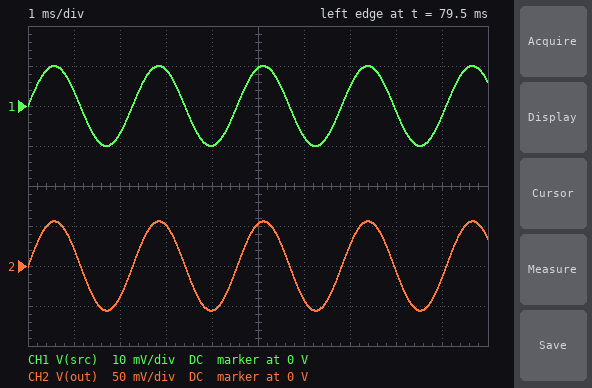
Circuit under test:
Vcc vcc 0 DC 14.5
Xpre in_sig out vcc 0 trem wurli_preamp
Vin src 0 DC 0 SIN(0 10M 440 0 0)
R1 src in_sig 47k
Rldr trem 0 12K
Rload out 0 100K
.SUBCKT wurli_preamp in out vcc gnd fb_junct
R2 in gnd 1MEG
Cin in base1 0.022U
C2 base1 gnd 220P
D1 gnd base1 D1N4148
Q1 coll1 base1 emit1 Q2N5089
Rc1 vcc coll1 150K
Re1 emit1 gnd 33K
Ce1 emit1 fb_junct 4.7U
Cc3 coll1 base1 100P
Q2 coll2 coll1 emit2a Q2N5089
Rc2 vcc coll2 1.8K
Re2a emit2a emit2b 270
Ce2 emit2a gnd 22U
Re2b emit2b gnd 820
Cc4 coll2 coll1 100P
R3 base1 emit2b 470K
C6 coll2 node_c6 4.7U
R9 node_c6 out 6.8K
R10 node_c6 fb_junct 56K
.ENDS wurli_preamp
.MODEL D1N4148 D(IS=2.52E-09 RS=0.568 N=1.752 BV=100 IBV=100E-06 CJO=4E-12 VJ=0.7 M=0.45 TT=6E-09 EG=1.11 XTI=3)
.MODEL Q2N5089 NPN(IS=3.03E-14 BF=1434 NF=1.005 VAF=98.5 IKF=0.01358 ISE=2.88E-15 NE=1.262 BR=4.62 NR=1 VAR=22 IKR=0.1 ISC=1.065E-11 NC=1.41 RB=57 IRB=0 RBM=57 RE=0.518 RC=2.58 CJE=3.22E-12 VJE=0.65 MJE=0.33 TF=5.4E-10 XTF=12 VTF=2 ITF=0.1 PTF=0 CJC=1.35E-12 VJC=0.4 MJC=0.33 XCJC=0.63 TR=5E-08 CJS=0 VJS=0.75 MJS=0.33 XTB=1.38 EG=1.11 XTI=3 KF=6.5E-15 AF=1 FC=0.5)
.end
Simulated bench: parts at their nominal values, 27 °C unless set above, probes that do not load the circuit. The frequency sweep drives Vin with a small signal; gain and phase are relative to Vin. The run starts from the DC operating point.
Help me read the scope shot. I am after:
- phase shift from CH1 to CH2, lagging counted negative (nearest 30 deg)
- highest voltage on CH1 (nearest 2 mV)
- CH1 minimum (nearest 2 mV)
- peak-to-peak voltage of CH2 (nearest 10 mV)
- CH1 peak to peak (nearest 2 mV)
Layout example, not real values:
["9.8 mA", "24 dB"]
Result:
["0 deg", "10 mV", "-10 mV", "110 mV", "20 mV"]
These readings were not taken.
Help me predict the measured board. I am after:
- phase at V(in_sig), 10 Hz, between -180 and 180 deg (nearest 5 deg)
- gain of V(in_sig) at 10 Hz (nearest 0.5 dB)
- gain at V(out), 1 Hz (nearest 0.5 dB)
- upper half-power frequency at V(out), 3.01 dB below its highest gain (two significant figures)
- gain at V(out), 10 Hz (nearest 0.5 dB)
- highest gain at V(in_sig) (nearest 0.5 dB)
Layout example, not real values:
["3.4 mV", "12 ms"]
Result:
["-5 deg", "-0.5 dB", "-22.0 dB", "8.8 kHz", "5.0 dB", "-0.5 dB"]
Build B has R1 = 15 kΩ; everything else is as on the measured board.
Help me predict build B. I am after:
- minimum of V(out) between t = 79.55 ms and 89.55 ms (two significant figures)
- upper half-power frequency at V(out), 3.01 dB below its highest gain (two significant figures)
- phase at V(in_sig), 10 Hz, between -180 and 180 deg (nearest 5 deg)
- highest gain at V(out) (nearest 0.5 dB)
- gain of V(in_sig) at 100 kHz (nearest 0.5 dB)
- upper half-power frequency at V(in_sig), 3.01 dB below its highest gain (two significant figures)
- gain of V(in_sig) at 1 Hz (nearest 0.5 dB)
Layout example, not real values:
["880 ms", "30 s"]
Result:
["-61 mV", "16 kHz", "0 deg", "16.5 dB", "-10.0 dB", "32 kHz", "0 dB"]
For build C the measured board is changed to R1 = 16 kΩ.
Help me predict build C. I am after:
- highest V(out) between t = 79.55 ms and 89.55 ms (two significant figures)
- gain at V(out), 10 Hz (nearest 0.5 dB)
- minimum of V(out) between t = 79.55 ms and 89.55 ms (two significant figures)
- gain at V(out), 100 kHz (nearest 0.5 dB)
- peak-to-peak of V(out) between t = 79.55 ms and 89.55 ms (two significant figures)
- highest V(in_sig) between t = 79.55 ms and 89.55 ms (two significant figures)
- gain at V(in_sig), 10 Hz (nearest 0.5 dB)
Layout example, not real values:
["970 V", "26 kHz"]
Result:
["61 mV", "5.5 dB", "-61 mV", "-5.0 dB", "120 mV", "9.5 mV", "0 dB"]
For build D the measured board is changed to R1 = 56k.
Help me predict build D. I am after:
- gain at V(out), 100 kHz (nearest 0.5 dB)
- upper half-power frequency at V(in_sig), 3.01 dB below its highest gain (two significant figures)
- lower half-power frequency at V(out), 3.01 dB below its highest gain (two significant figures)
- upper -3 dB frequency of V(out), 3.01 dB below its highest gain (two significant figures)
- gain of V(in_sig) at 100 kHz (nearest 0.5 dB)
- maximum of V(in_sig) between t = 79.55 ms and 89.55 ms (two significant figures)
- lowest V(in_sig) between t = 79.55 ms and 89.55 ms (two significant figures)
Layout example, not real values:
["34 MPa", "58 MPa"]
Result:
["-15.5 dB", "8.1 kHz", "17 Hz", "7.9 kHz", "-21.0 dB", "8.5 mV", "-8.5 mV"]
